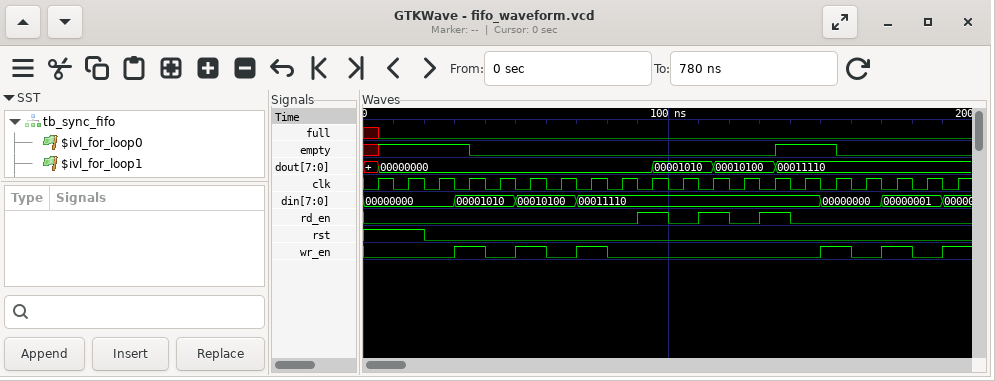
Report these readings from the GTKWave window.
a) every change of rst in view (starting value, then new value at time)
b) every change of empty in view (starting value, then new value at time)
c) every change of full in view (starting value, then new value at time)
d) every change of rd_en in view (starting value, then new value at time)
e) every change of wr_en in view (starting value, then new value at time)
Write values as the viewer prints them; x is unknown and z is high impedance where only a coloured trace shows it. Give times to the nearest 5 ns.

1, 0 at 20 ns
x, 1 at 5 ns, 0 at 35 ns, 1 at 135 ns, 0 at 155 ns
x, 0 at 5 ns
0, 1 at 90 ns, 0 at 100 ns, 1 at 110 ns, 0 at 120 ns, 1 at 130 ns, 0 at 140 ns
0, 1 at 30 ns, 0 at 40 ns, 1 at 50 ns, 0 at 60 ns, 1 at 70 ns, 0 at 80 ns, 1 at 150 ns, 0 at 160 ns, 1 at 170 ns, 0 at 180 ns, 1 at 190 ns
